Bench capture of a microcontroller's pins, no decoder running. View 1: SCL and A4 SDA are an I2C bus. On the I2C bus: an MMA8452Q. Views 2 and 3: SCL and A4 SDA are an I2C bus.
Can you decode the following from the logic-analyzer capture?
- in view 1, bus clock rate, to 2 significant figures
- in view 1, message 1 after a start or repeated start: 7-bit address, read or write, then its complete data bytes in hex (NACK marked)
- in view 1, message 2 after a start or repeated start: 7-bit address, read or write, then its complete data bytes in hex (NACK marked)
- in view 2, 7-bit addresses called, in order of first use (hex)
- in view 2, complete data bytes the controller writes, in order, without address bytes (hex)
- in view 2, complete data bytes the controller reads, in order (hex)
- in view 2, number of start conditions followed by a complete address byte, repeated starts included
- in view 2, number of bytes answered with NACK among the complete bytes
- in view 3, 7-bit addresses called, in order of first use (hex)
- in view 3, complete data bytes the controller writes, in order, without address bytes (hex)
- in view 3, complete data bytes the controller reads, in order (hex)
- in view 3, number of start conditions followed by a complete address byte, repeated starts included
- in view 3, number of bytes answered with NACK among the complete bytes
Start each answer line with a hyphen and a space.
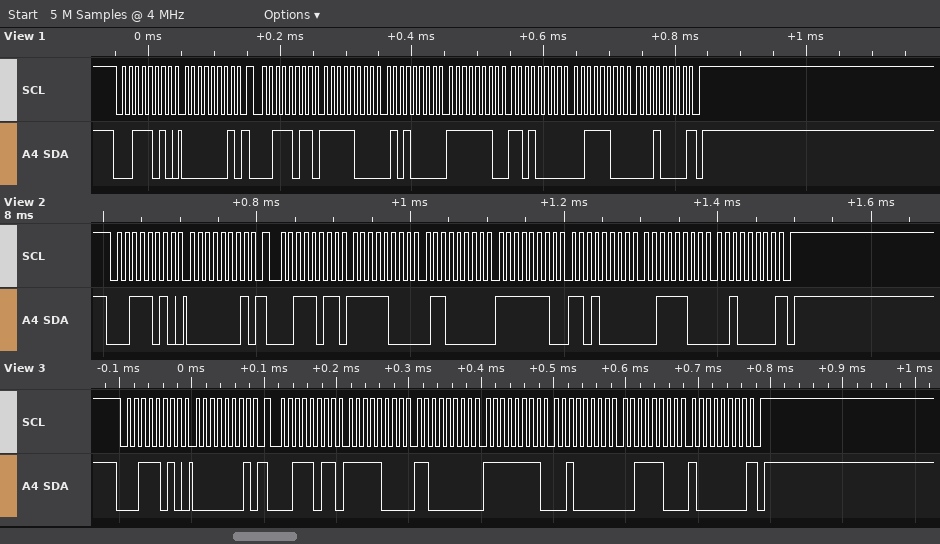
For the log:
- 100 kHz
- 0x1D write: 01
- 0x1D read: F8 50 FE D0 3C 10 NACK
- 0x1D
- 01
- F8 60 FE D0 3C 20
- 2
- 1
- 0x1D
- 01
- F8 C0 FF 20 3C 80
- 2
- 1
